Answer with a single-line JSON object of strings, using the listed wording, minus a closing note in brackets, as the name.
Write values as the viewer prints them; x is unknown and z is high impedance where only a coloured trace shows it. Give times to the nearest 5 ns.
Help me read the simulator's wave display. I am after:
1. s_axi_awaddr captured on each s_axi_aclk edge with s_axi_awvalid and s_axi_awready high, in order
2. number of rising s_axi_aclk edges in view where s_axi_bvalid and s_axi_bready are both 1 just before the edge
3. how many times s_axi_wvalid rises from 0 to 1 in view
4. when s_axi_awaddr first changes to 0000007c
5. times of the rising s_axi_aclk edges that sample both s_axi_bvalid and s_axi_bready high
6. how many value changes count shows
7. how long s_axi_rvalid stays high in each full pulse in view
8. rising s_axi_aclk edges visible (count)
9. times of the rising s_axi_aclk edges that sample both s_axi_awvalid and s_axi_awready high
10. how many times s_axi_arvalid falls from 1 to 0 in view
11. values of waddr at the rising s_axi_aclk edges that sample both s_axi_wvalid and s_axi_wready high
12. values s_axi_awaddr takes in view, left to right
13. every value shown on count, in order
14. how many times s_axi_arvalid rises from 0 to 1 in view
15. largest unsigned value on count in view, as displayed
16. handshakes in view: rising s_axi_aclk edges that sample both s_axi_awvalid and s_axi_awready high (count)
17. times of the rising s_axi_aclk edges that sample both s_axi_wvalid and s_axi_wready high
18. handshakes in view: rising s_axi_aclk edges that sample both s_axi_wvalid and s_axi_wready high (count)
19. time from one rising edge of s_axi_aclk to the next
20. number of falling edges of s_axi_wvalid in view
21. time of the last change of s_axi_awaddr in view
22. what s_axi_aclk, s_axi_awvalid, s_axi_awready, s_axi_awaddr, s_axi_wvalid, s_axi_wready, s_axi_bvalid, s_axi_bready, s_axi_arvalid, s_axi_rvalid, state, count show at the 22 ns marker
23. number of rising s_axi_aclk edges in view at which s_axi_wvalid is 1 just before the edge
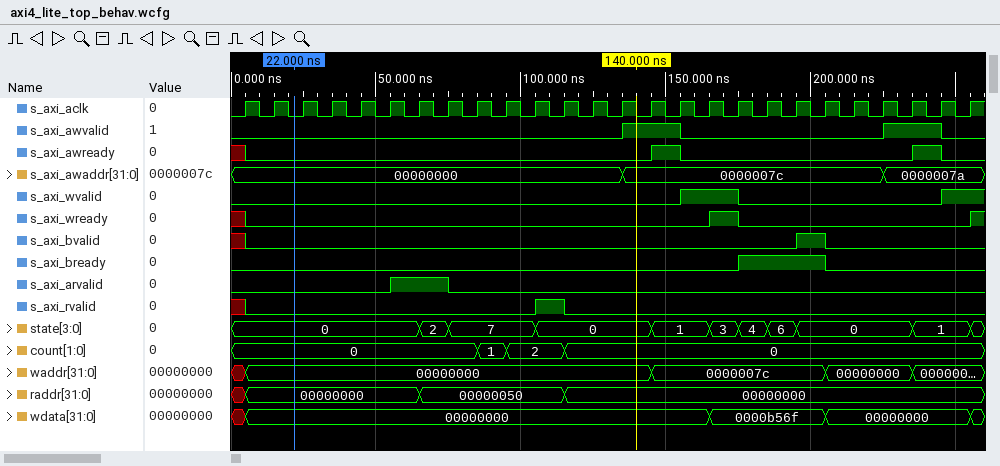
{"s_axi_awaddr captured on each s_axi_aclk edge with s_axi_awvalid and s_axi_awready high, in order": "0000007c, 0000007a", "number of rising s_axi_aclk edges in view where s_axi_bvalid and s_axi_bready are both 1 just before the edge": "1", "how many times s_axi_wvalid rises from 0 to 1 in view": "2", "when s_axi_awaddr first changes to 0000007c": "135 ns", "times of the rising s_axi_aclk edges that sample both s_axi_bvalid and s_axi_bready high": "205 ns", "how many value changes count shows": "3", "how long s_axi_rvalid stays high in each full pulse in view": "10 ns", "rising s_axi_aclk edges visible": "26", "times of the rising s_axi_aclk edges that sample both s_axi_awvalid and s_axi_awready high": "155 ns, 245 ns", "how many times s_axi_arvalid falls from 1 to 0 in view": "1", "values of waddr at the rising s_axi_aclk edges that sample both s_axi_wvalid and s_axi_wready high": "0000007c", "values s_axi_awaddr takes in view, left to right": "00000000, 0000007c, 0000007a", "every value shown on count, in order": "0, 1, 2, 0", "how many times s_axi_arvalid rises from 0 to 1 in view": "1", "largest unsigned value on count in view, as displayed": "2", "handshakes in view: rising s_axi_aclk edges that sample both s_axi_awvalid and s_axi_awready high": "2", "times of the rising s_axi_aclk edges that sample both s_axi_wvalid and s_axi_wready high": "175 ns", "handshakes in view: rising s_axi_aclk edges that sample both s_axi_wvalid and s_axi_wready high": "1", "time from one rising edge of s_axi_aclk to the next": "10 ns", "number of falling edges of s_axi_wvalid in view": "1", "time of the last change of s_axi_awaddr in view": "225 ns", "what s_axi_aclk, s_axi_awvalid, s_axi_awready, s_axi_awaddr, s_axi_wvalid, s_axi_wready, s_axi_bvalid, s_axi_bready, s_axi_arvalid, s_axi_rvalid, state, count show at the 22 ns marker": "s_axi_aclk=0, s_axi_awvalid=0, s_axi_awready=0, s_axi_awaddr=00000000, s_axi_wvalid=0, s_axi_wready=0, s_axi_bvalid=0, s_axi_bready=0, s_axi_arvalid=0, s_axi_rvalid=0, state=0, count=0", "number of rising s_axi_aclk edges in view at which s_axi_wvalid is 1 just before the edge": "3"}
